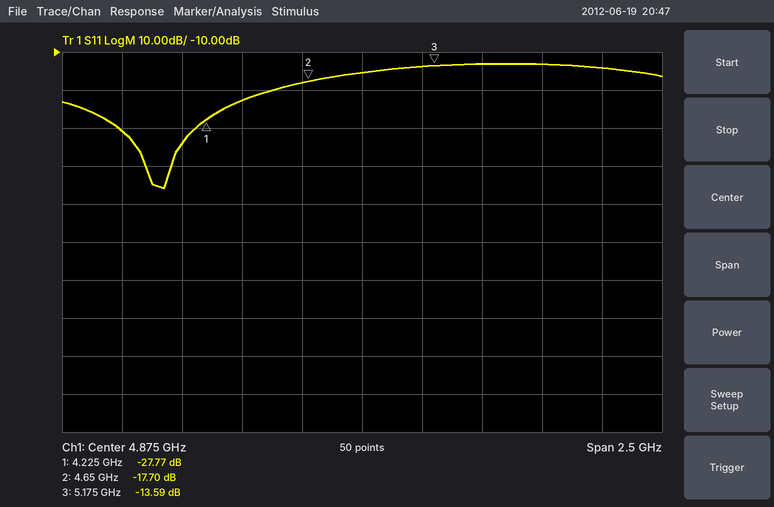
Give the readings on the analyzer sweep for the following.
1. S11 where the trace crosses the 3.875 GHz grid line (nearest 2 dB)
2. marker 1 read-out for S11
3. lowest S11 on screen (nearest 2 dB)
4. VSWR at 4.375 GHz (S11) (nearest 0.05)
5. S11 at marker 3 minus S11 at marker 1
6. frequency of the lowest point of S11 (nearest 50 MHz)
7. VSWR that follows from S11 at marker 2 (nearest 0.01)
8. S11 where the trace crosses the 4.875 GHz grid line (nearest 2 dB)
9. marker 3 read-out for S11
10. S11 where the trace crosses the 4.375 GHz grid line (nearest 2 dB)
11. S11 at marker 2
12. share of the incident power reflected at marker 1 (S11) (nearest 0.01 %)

-30 dB
-27.77 dB
-46 dB
1.15
14.18 dB
4.05 GHz
1.30
-16 dB
-13.59 dB
-22 dB
-17.70 dB
0.17 %
